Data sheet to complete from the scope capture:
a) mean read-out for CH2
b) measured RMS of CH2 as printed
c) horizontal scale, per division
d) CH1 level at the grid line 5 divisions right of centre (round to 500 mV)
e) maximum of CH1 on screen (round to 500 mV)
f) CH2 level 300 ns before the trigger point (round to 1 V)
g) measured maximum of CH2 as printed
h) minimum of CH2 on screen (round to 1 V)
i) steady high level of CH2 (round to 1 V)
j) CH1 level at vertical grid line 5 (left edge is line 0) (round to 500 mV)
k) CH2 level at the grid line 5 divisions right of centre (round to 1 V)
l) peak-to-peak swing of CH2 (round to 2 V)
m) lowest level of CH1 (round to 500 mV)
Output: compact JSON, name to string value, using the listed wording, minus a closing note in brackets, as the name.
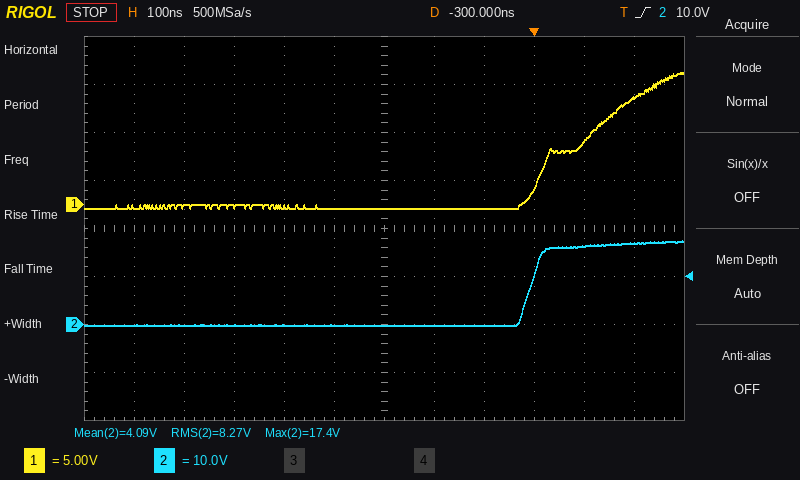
{"mean read-out for CH2": "4.09 V", "measured RMS of CH2 as printed": "8.27 V", "horizontal scale, per division": "100 ns", "CH1 level at the grid line 5 divisions right of centre": "11.0 V", "maximum of CH1 on screen": "14.0 V", "CH2 level 300 ns before the trigger point": "0 V", "measured maximum of CH2 as printed": "17.4 V", "minimum of CH2 on screen": "0 V", "steady high level of CH2": "17 V", "CH1 level at vertical grid line 5 (left edge is line 0)": "-500 mV", "CH2 level at the grid line 5 divisions right of centre": "17 V", "peak-to-peak swing of CH2": "18 V", "lowest level of CH1": "-500 mV"}
